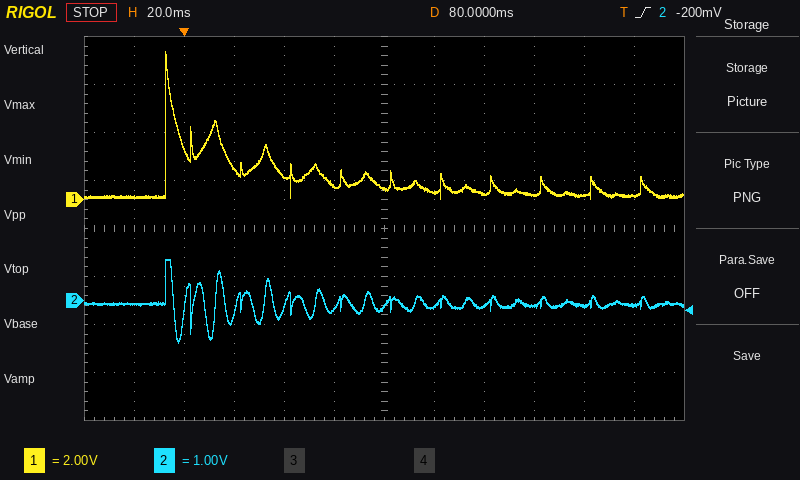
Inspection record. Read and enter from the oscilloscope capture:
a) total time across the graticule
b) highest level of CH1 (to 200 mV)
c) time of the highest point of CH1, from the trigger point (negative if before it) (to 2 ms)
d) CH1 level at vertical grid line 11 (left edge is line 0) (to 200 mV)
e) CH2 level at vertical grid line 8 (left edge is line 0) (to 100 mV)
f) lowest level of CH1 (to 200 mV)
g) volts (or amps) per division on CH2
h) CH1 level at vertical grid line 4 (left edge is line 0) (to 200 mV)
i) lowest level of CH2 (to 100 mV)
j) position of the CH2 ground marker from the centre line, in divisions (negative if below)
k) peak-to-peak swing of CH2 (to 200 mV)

240 ms
6.2 V
-8 ms
200 mV
-100 mV
0.0 V
1 V
1.0 V
-900 mV
-1.5 div
1.8 V
